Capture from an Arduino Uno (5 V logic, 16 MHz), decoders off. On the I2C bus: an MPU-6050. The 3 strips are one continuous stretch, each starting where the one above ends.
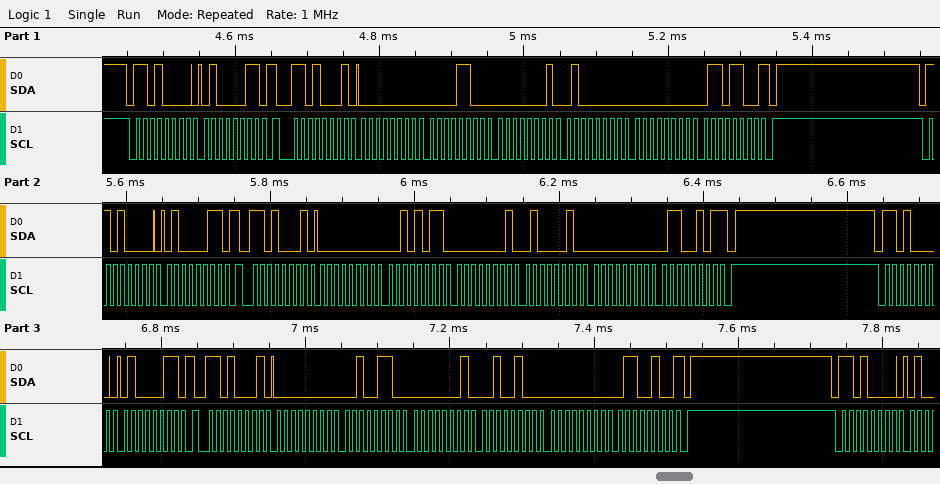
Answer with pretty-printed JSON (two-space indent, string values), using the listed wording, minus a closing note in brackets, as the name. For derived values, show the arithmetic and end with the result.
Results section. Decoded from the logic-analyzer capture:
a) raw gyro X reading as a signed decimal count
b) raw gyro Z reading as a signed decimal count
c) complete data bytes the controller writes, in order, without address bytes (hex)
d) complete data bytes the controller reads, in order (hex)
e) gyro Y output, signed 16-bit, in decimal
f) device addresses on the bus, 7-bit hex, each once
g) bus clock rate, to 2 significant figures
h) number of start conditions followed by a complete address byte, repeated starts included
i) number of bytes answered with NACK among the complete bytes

{
  "raw gyro X reading as a signed decimal count": "0x000C = 12",
  "raw gyro Z reading as a signed decimal count": "0x006C = 108",
  "complete data bytes the controller writes, in order, without address bytes": "43 43 43",
  "complete data bytes the controller reads, in order": "00 0C 01 40 00 6C 00 2B 01 42 00 65 00 26 01 24 00 64",
  "gyro Y output, signed 16-bit, in decimal": "0x0140 = 320",
  "device addresses on the bus, 7-bit hex, each once": "0x68",
  "bus clock rate, to 2 significant figures": "100 kHz",
  "number of start conditions followed by a complete address byte, repeated starts included": "7",
  "number of bytes answered with NACK among the complete bytes": "3"
}
